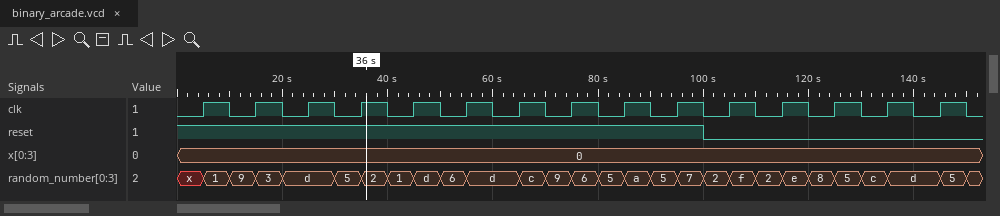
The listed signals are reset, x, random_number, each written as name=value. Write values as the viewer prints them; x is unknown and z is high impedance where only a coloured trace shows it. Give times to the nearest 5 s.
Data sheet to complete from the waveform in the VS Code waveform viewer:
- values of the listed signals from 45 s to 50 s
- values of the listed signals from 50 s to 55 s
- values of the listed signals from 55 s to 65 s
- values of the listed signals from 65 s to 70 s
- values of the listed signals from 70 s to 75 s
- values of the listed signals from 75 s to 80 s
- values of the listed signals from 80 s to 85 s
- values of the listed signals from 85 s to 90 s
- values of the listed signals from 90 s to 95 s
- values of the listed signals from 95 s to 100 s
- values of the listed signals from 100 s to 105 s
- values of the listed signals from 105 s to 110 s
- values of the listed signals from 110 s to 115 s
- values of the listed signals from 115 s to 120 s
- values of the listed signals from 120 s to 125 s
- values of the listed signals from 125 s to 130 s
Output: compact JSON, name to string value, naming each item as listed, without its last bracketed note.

{"values of the listed signals from 45 s to 50 s": "reset=1, x=0, random_number=d", "values of the listed signals from 50 s to 55 s": "reset=1, x=0, random_number=6", "values of the listed signals from 55 s to 65 s": "reset=1, x=0, random_number=d", "values of the listed signals from 65 s to 70 s": "reset=1, x=0, random_number=c", "values of the listed signals from 70 s to 75 s": "reset=1, x=0, random_number=9", "values of the listed signals from 75 s to 80 s": "reset=1, x=0, random_number=6", "values of the listed signals from 80 s to 85 s": "reset=1, x=0, random_number=5", "values of the listed signals from 85 s to 90 s": "reset=1, x=0, random_number=a", "values of the listed signals from 90 s to 95 s": "reset=1, x=0, random_number=5", "values of the listed signals from 95 s to 100 s": "reset=1, x=0, random_number=7", "values of the listed signals from 100 s to 105 s": "reset=0, x=0, random_number=2", "values of the listed signals from 105 s to 110 s": "reset=0, x=0, random_number=f", "values of the listed signals from 110 s to 115 s": "reset=0, x=0, random_number=2", "values of the listed signals from 115 s to 120 s": "reset=0, x=0, random_number=e", "values of the listed signals from 120 s to 125 s": "reset=0, x=0, random_number=8", "values of the listed signals from 125 s to 130 s": "reset=0, x=0, random_number=5"}
